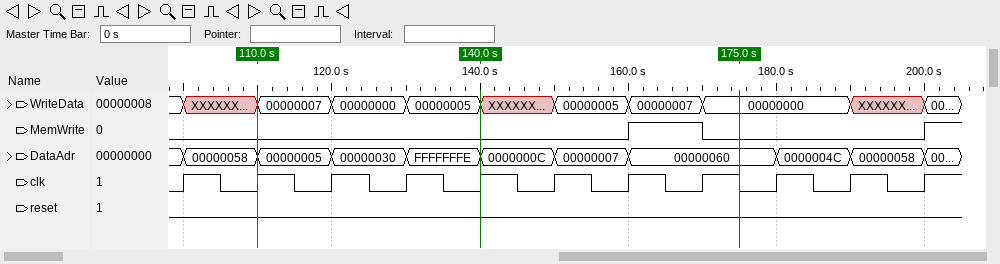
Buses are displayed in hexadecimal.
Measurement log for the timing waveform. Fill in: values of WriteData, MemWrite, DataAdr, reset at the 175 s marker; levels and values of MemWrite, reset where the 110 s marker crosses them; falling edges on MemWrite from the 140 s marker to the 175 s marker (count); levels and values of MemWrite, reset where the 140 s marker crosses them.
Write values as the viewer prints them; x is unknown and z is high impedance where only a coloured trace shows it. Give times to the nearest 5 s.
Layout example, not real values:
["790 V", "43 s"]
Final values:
["WriteData=00000000, MemWrite=0, DataAdr=00000060, reset=0", "MemWrite=0, reset=0", "1", "MemWrite=0, reset=0"]
